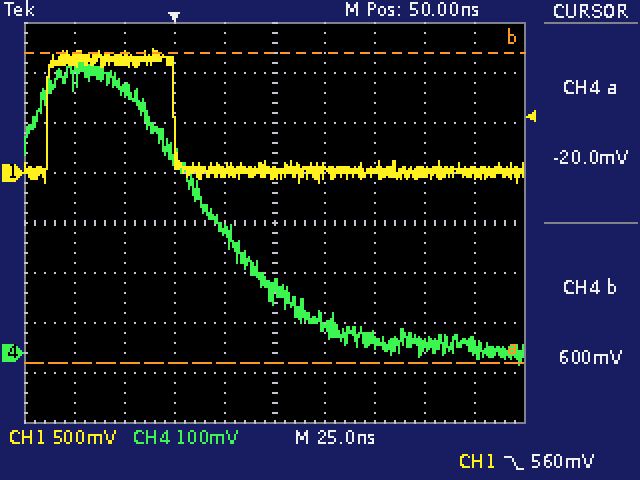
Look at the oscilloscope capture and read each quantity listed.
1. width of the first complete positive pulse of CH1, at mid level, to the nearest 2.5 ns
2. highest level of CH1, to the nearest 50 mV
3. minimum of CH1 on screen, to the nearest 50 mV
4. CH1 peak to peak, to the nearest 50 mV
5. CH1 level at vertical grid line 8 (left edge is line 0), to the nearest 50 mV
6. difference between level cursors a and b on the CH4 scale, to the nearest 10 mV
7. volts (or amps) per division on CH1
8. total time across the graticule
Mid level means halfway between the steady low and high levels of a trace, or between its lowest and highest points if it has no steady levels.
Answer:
62.5 ns
1.25 V
-100 mV
1.35 V
0 mV
620 mV
500 mV
250 ns
